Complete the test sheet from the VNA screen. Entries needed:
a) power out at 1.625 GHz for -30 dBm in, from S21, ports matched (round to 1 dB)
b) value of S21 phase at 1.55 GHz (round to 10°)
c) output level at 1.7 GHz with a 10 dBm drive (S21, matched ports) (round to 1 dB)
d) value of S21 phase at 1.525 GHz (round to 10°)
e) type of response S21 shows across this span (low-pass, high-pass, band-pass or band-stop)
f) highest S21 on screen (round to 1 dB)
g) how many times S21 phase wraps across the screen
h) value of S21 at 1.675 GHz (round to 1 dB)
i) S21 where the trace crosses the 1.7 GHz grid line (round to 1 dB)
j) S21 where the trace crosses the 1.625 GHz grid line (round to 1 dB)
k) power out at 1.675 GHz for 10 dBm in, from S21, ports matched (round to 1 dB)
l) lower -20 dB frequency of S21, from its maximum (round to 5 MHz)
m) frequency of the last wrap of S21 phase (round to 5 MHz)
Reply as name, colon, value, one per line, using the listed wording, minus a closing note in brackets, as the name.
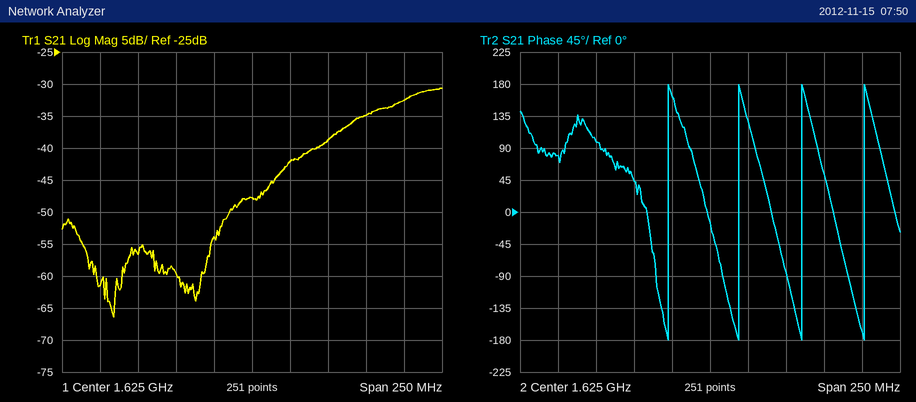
power out at 1.625 GHz for -30 dBm in, from S21, ports matched: -78 dBm
value of S21 phase at 1.55 GHz: 100°
output level at 1.7 GHz with a 10 dBm drive (S21, matched ports): -25 dBm
value of S21 phase at 1.525 GHz: 80°
type of response S21 shows across this span: high-pass
highest S21 on screen: -31 dB
how many times S21 phase wraps across the screen: 4
value of S21 at 1.675 GHz: -39 dB
S21 where the trace crosses the 1.7 GHz grid line: -35 dB
S21 where the trace crosses the 1.625 GHz grid line: -48 dB
power out at 1.675 GHz for 10 dBm in, from S21, ports matched: -29 dBm
lower -20 dB frequency of S21, from its maximum: 1.610 GHz
frequency of the last wrap of S21 phase: 1.725 GHz
